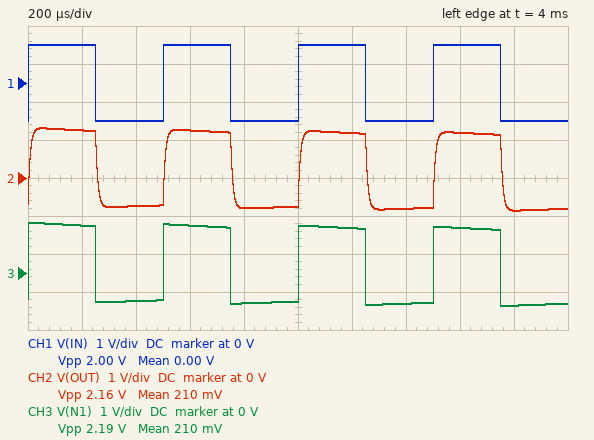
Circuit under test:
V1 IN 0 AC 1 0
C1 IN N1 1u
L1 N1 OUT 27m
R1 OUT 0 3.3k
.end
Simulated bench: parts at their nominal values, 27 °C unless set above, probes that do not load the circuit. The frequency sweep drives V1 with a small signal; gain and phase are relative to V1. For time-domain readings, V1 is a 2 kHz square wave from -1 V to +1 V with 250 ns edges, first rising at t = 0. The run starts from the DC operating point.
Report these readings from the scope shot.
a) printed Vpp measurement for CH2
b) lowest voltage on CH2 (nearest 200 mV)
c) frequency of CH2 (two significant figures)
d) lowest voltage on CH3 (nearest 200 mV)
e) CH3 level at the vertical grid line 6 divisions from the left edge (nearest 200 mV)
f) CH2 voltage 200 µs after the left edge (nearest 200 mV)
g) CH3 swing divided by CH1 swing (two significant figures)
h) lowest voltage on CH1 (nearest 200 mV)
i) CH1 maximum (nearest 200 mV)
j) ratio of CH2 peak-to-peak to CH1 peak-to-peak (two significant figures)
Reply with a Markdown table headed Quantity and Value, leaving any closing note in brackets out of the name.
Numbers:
| Quantity | Value |
|---|---|
| printed Vpp measurement for CH2 | 2.16 V |
| lowest voltage on CH2 | -800 mV |
| frequency of CH2 | 2.0 kHz |
| lowest voltage on CH3 | -800 mV |
| CH3 level at the vertical grid line 6 divisions from the left edge | 1.2 V |
| CH2 voltage 200 µs after the left edge | 1.2 V |
| CH3 swing divided by CH1 swing | 1.1 |
| lowest voltage on CH1 | -1.0 V |
| CH1 maximum | 1.0 V |
| ratio of CH2 peak-to-peak to CH1 peak-to-peak | 1.1 |
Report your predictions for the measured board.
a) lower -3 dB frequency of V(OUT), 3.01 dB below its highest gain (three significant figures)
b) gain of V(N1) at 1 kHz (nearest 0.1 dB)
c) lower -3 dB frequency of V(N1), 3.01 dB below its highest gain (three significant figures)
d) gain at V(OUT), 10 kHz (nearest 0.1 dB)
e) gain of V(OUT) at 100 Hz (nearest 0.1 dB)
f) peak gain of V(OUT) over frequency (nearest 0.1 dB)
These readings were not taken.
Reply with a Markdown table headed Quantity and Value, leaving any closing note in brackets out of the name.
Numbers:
| Quantity | Value |
|---|---|
| lower -3 dB frequency of V(OUT), 3.01 dB below its highest gain | 48.1 Hz |
| gain of V(N1) at 1 kHz | 0 dB |
| lower -3 dB frequency of V(N1), 3.01 dB below its highest gain | 48.3 Hz |
| gain at V(OUT), 10 kHz | -1.0 dB |
| gain of V(OUT) at 100 Hz | -0.9 dB |
| peak gain of V(OUT) over frequency | 0 dB |
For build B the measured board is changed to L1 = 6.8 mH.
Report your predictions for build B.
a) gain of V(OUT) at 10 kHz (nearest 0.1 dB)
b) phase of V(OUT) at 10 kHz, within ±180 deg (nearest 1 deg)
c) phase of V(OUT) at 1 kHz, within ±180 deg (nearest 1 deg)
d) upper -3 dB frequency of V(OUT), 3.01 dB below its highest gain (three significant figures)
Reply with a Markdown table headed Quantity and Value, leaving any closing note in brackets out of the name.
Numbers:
| Quantity | Value |
|---|---|
| gain of V(OUT) at 10 kHz | -0.1 dB |
| phase of V(OUT) at 10 kHz, within ±180 deg | -7 deg |
| phase of V(OUT) at 1 kHz, within ±180 deg | 2 deg |
| upper -3 dB frequency of V(OUT), 3.01 dB below its highest gain | 77.3 kHz |
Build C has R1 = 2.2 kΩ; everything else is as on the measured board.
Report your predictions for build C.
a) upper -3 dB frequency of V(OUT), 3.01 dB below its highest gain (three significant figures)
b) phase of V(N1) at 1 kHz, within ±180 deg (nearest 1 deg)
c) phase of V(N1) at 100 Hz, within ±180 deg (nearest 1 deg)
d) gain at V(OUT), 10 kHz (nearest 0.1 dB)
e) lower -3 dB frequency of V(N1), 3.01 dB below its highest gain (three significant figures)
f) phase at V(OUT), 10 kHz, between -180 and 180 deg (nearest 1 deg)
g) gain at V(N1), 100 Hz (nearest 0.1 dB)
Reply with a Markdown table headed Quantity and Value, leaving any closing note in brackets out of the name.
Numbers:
| Quantity | Value |
|---|---|
| upper -3 dB frequency of V(OUT), 3.01 dB below its highest gain | 13.0 kHz |
| phase of V(N1) at 1 kHz, within ±180 deg | 4 deg |
| phase of V(N1) at 100 Hz, within ±180 deg | 36 deg |
| gain at V(OUT), 10 kHz | -2.0 dB |
| lower -3 dB frequency of V(N1), 3.01 dB below its highest gain | 72.7 Hz |
| phase at V(OUT), 10 kHz, between -180 and 180 deg | -37 deg |
| gain at V(N1), 100 Hz | -1.8 dB |
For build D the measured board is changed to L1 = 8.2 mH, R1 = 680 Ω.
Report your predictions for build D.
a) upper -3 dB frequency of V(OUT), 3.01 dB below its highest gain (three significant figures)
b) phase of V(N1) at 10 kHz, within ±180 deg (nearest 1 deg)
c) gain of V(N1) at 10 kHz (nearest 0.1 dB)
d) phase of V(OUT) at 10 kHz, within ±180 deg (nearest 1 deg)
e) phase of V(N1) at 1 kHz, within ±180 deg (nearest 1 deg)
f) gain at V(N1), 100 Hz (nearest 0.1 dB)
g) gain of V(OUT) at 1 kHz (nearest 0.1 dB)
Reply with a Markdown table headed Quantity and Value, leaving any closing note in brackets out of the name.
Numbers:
| Quantity | Value |
|---|---|
| upper -3 dB frequency of V(OUT), 3.01 dB below its highest gain | 13.4 kHz |
| phase of V(N1) at 10 kHz, within ±180 deg | 1 deg |
| gain of V(N1) at 10 kHz | 0.1 dB |
| phase of V(OUT) at 10 kHz, within ±180 deg | -36 deg |
| phase of V(N1) at 1 kHz, within ±180 deg | 13 deg |
| gain at V(N1), 100 Hz | -8.1 dB |
| gain of V(OUT) at 1 kHz | -0.1 dB |
